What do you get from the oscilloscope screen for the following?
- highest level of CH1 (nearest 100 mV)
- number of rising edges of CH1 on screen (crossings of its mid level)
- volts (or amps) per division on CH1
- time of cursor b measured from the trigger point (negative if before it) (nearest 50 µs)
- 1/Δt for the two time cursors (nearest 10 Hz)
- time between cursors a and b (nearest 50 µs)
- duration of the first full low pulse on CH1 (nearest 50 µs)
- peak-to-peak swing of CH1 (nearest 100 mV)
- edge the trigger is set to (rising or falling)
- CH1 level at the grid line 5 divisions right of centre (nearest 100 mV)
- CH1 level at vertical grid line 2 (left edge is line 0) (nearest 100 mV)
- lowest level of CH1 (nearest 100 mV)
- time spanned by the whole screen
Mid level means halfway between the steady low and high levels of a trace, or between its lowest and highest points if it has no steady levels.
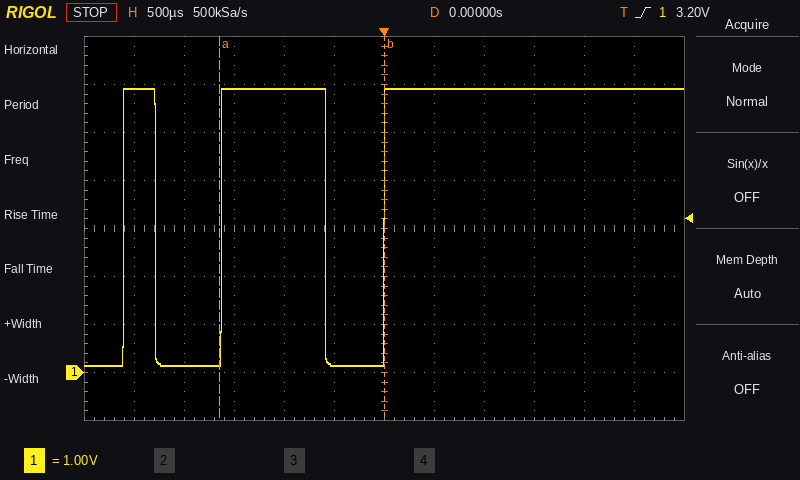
5.9 V
3
1 V
0 µs
610 Hz
1.65 ms
650 µs
5.8 V
rising
5.9 V
100 mV
100 mV
6 ms
